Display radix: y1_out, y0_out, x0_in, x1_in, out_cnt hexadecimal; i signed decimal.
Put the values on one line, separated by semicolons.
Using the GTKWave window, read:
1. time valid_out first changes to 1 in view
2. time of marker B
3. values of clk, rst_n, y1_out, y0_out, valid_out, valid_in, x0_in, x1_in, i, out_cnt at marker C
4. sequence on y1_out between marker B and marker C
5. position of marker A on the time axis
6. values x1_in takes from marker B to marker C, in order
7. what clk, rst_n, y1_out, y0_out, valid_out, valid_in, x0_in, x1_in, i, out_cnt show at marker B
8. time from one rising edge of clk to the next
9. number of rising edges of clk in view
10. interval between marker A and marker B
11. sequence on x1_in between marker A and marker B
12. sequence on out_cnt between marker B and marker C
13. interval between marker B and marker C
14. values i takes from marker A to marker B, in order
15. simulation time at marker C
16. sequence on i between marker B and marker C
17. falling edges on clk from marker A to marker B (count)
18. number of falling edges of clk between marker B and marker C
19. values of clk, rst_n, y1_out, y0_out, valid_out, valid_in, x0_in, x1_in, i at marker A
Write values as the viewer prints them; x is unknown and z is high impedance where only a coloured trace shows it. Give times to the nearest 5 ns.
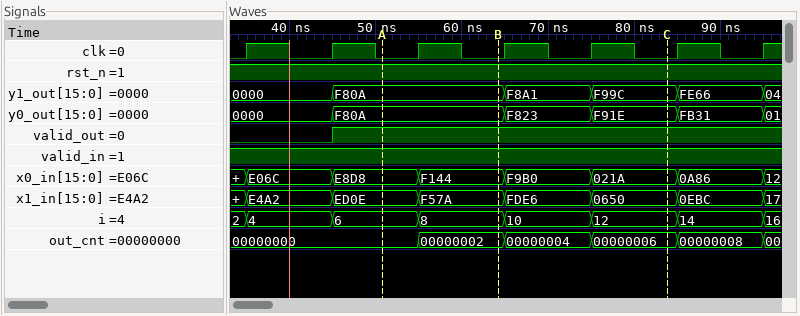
45 ns; 65 ns; clk=0, rst_n=1, y1_out=F99C, y0_out=F91E, valid_out=1, valid_in=1, x0_in=021A, x1_in=0650, i=12, out_cnt=00000006; F80A, F8A1, F99C; 50 ns; F57A, FDE6, 0650; clk=0, rst_n=1, y1_out=F80A, y0_out=F80A, valid_out=1, valid_in=1, x0_in=F144, x1_in=F57A, i=8, out_cnt=00000002; 10 ns; 7; 15 ns; ED0E, F57A; 00000002, 00000004, 00000006; 20 ns; 6, 8; 85 ns; 8, 10, 12; 1; 2; clk=0, rst_n=1, y1_out=F80A, y0_out=F80A, valid_out=1, valid_in=1, x0_in=E8D8, x1_in=ED0E, i=6
